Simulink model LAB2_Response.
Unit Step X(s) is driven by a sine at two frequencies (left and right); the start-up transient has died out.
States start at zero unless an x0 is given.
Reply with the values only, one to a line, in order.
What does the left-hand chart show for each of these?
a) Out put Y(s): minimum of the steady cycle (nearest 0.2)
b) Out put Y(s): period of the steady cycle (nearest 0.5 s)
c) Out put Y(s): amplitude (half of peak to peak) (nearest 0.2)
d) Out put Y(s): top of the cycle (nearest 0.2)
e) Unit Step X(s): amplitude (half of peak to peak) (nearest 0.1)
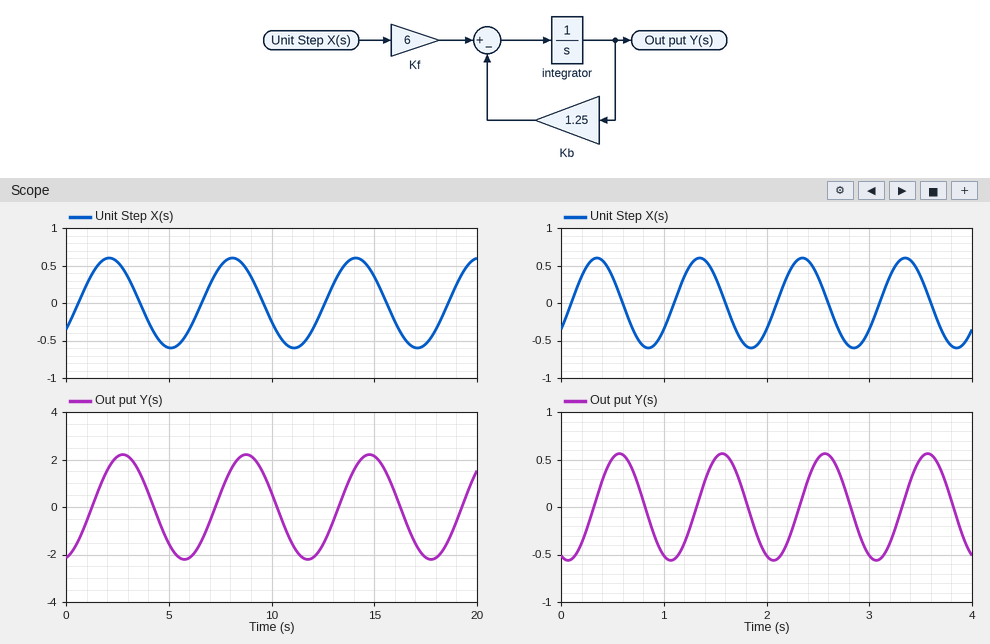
-2.2
6.0 s
2.2
2.2
0.6
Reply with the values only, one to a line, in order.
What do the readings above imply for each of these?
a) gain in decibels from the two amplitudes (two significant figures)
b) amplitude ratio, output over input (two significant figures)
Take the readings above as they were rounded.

11 dB
3.7
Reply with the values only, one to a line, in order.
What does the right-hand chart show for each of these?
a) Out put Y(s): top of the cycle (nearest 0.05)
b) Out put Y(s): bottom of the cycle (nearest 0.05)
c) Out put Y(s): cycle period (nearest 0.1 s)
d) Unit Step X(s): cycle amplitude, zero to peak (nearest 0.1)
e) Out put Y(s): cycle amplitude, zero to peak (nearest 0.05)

0.55
-0.55
1.0 s
0.6
0.55
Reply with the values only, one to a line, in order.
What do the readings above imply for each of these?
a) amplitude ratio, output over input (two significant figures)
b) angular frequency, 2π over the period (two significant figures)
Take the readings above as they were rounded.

0.92
6.3 rad/s
